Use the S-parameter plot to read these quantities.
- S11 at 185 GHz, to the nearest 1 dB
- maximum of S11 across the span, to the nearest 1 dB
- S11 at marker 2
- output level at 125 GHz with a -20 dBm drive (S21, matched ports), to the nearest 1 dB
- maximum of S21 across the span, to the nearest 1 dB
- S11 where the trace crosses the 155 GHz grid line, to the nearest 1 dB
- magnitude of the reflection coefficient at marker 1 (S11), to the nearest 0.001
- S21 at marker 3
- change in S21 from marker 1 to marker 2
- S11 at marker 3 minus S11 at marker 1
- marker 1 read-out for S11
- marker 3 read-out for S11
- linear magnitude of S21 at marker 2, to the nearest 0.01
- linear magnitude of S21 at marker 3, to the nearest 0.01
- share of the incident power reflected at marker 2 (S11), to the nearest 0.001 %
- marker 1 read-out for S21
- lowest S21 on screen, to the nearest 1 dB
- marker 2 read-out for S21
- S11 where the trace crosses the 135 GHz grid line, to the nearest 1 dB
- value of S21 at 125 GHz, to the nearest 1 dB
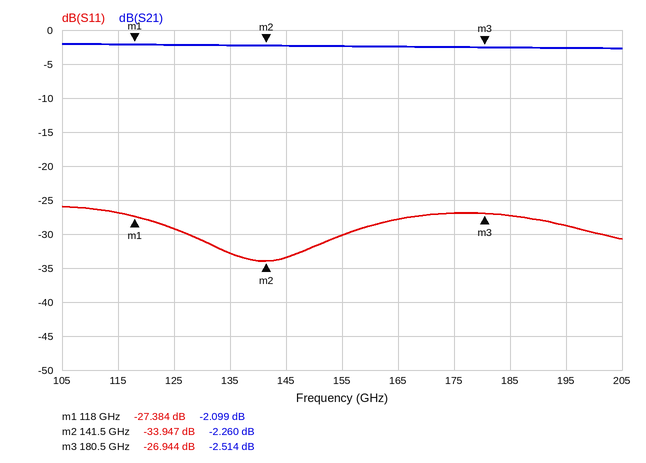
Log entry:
-27 dB
-26 dB
-33.947 dB
-22 dBm
-2 dB
-30 dB
0.043
-2.514 dB
-0.161 dB
0.440 dB
-27.384 dB
-26.944 dB
0.77
0.75
0.040 %
-2.099 dB
-3 dB
-2.260 dB
-33 dB
-2 dB
